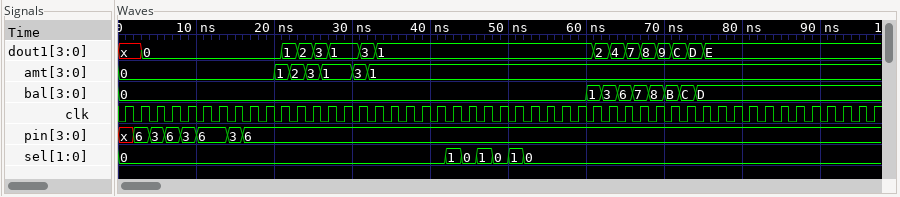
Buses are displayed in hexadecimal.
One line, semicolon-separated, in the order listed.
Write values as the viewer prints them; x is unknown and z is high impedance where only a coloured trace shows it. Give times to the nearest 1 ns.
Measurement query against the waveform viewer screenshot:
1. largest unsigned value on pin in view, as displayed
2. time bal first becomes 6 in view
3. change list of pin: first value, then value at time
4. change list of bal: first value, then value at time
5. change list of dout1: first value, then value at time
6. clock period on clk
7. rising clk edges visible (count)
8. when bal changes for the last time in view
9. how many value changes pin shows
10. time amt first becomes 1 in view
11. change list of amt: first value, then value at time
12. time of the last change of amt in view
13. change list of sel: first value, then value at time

6; 64 ns; x, 6 at 2 ns, 3 at 4 ns, 6 at 6 ns, 3 at 8 ns, 6 at 10 ns, 3 at 14 ns, 6 at 16 ns; 0, 1 at 60 ns, 3 at 62 ns, 6 at 64 ns, 7 at 66 ns, 8 at 68 ns, B at 70 ns, C at 72 ns, D at 74 ns; x, 0 at 3 ns, 1 at 21 ns, 2 at 23 ns, 3 at 25 ns, 1 at 27 ns, 3 at 31 ns, 1 at 33 ns, 2 at 61 ns, 4 at 63 ns, 7 at 65 ns, 8 at 67 ns, 9 at 69 ns, C at 71 ns, D at 73 ns, E at 75 ns; 2 ns; 49; 74 ns; 7; 20 ns; 0, 1 at 20 ns, 2 at 22 ns, 3 at 24 ns, 1 at 26 ns, 3 at 30 ns, 1 at 32 ns; 32 ns; 0, 1 at 42 ns, 0 at 44 ns, 1 at 46 ns, 0 at 48 ns, 1 at 50 ns, 0 at 52 ns
